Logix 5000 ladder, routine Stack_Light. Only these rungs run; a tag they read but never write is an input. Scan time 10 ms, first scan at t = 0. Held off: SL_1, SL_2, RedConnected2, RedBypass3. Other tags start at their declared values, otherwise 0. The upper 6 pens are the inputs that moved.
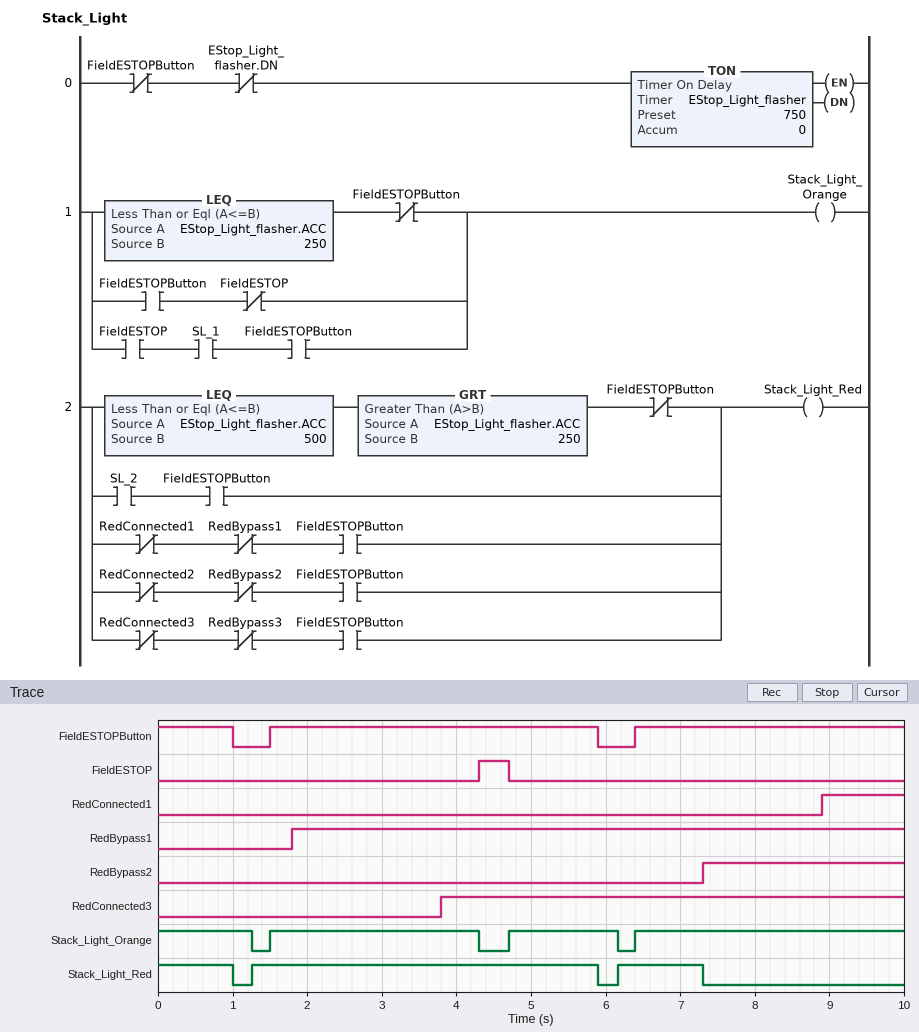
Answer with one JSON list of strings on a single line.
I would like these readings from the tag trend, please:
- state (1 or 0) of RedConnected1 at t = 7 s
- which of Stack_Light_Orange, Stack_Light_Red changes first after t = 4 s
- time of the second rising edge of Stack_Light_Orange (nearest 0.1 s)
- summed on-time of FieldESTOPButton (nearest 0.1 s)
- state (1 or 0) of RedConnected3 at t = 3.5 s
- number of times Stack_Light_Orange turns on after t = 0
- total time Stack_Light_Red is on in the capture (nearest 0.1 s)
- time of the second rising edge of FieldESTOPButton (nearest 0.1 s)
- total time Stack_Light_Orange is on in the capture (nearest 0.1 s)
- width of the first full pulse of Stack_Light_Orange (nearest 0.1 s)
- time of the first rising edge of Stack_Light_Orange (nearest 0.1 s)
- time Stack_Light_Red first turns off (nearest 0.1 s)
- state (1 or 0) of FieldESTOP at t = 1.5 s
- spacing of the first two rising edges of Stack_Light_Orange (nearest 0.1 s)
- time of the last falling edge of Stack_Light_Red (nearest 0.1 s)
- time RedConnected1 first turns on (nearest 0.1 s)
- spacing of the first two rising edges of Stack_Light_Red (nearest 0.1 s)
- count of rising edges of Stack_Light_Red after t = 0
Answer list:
["0", "Stack_Light_Orange", "4.7 s", "9.0 s", "0", "3", "6.8 s", "6.4 s", "9.1 s", "2.8 s", "1.5 s", "1.0 s", "0", "3.2 s", "7.3 s", "8.9 s", "4.9 s", "2"]
